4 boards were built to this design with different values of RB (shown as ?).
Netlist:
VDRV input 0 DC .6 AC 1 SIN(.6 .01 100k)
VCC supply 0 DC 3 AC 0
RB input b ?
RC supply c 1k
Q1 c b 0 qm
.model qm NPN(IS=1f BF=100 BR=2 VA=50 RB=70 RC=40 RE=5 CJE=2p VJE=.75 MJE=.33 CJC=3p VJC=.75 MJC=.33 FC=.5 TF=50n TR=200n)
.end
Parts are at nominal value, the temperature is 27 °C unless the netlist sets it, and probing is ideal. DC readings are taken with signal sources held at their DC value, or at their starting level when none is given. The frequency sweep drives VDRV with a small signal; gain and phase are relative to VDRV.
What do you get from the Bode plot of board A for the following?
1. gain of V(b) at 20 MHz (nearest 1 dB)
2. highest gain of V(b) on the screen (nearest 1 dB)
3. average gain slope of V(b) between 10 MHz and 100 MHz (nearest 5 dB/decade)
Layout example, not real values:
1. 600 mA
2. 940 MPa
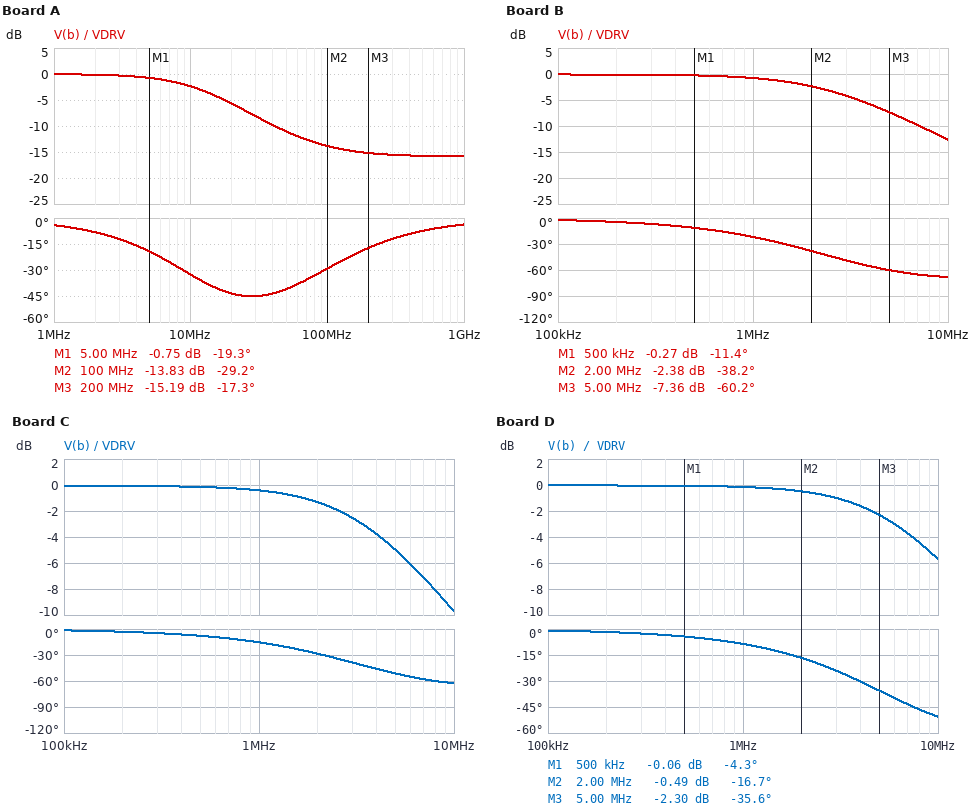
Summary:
1. -6 dB
2. 0 dB
3. -10 dB/decade
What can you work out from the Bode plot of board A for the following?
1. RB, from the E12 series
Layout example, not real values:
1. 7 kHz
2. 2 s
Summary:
1. 390 Ω
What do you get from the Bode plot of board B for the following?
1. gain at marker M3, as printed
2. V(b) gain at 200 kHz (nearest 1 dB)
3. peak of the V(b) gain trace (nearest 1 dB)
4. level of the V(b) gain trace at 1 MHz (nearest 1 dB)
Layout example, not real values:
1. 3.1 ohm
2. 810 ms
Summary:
1. -7.36 dB
2. 0 dB
3. 0 dB
4. -1 dB
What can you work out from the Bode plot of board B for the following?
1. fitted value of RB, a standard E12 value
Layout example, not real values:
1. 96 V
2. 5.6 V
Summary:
1. 2.2 kΩ
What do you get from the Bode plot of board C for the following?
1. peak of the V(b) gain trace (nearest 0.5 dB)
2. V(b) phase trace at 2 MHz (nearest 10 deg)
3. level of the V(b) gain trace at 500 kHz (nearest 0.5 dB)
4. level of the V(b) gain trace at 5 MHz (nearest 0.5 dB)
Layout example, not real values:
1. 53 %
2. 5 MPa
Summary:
1. 0 dB
2. -30 deg
3. 0 dB
4. -5.0 dB
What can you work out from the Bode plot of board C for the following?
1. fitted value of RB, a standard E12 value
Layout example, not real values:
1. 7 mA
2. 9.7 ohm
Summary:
1. 1.5 kΩ
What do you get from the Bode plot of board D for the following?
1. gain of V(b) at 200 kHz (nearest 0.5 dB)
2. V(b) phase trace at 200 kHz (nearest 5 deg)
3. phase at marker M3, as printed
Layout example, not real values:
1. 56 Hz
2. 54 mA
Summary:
1. 0 dB
2. 0 deg
3. -35.6 deg
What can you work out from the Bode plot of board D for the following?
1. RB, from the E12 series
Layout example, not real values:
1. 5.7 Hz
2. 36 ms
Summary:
1. 820 Ω
